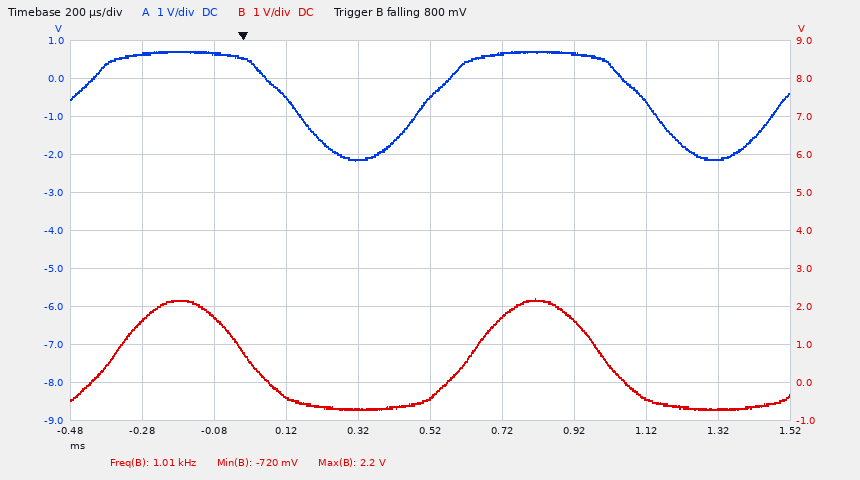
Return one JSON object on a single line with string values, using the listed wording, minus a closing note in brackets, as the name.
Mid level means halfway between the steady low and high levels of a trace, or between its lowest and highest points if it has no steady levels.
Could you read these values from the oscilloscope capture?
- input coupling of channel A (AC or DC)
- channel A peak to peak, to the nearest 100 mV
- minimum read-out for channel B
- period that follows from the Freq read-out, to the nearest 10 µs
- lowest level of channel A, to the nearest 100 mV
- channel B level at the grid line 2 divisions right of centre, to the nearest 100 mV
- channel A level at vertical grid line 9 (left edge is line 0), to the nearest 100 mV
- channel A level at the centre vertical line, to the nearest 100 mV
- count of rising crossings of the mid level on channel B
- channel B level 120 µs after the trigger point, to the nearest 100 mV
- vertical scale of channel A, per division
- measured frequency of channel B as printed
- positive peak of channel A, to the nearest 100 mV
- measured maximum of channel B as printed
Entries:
{"input coupling of channel A": "DC", "channel A peak to peak, to the nearest 100 mV": "2.9 V", "minimum read-out for channel B": "-720 mV", "period that follows from the Freq read-out, to the nearest 10 µs": "990 µs", "lowest level of channel A, to the nearest 100 mV": "-2.2 V", "channel B level at the grid line 2 divisions right of centre, to the nearest 100 mV": "1.6 V", "channel A level at vertical grid line 9 (left edge is line 0), to the nearest 100 mV": "-2.1 V", "channel A level at the centre vertical line, to the nearest 100 mV": "-500 mV", "count of rising crossings of the mid level on channel B": "2", "channel B level 120 µs after the trigger point, to the nearest 100 mV": "-400 mV", "vertical scale of channel A, per division": "1 V", "measured frequency of channel B as printed": "1.01 kHz", "positive peak of channel A, to the nearest 100 mV": "700 mV", "measured maximum of channel B as printed": "2.2 V"}
